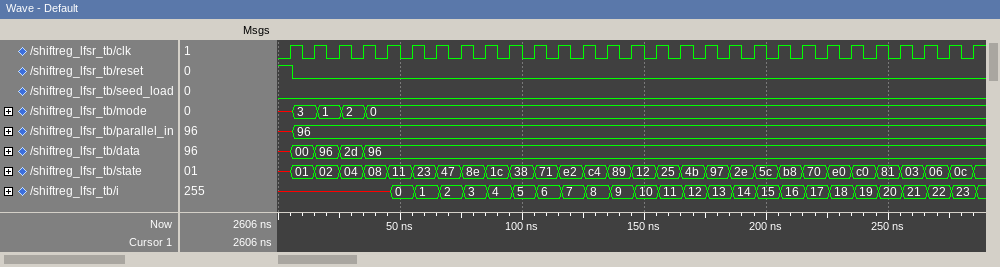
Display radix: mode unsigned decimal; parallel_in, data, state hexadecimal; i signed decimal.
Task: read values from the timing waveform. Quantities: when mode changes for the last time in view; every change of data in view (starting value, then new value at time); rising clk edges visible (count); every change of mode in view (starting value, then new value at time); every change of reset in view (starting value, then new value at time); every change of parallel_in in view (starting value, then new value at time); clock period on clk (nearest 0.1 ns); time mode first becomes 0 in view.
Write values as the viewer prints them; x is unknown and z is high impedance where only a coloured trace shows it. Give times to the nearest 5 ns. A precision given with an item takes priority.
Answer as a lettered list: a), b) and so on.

a) 35 ns
b) x, 00 at 5 ns, 96 at 15 ns, 2d at 25 ns, 96 at 35 ns
c) 29
d) x, 3 at 5 ns, 1 at 15 ns, 2 at 25 ns, 0 at 35 ns
e) 1, 0 at 5 ns
f) x, 96 at 5 ns
g) 10 ns
h) 35 ns
